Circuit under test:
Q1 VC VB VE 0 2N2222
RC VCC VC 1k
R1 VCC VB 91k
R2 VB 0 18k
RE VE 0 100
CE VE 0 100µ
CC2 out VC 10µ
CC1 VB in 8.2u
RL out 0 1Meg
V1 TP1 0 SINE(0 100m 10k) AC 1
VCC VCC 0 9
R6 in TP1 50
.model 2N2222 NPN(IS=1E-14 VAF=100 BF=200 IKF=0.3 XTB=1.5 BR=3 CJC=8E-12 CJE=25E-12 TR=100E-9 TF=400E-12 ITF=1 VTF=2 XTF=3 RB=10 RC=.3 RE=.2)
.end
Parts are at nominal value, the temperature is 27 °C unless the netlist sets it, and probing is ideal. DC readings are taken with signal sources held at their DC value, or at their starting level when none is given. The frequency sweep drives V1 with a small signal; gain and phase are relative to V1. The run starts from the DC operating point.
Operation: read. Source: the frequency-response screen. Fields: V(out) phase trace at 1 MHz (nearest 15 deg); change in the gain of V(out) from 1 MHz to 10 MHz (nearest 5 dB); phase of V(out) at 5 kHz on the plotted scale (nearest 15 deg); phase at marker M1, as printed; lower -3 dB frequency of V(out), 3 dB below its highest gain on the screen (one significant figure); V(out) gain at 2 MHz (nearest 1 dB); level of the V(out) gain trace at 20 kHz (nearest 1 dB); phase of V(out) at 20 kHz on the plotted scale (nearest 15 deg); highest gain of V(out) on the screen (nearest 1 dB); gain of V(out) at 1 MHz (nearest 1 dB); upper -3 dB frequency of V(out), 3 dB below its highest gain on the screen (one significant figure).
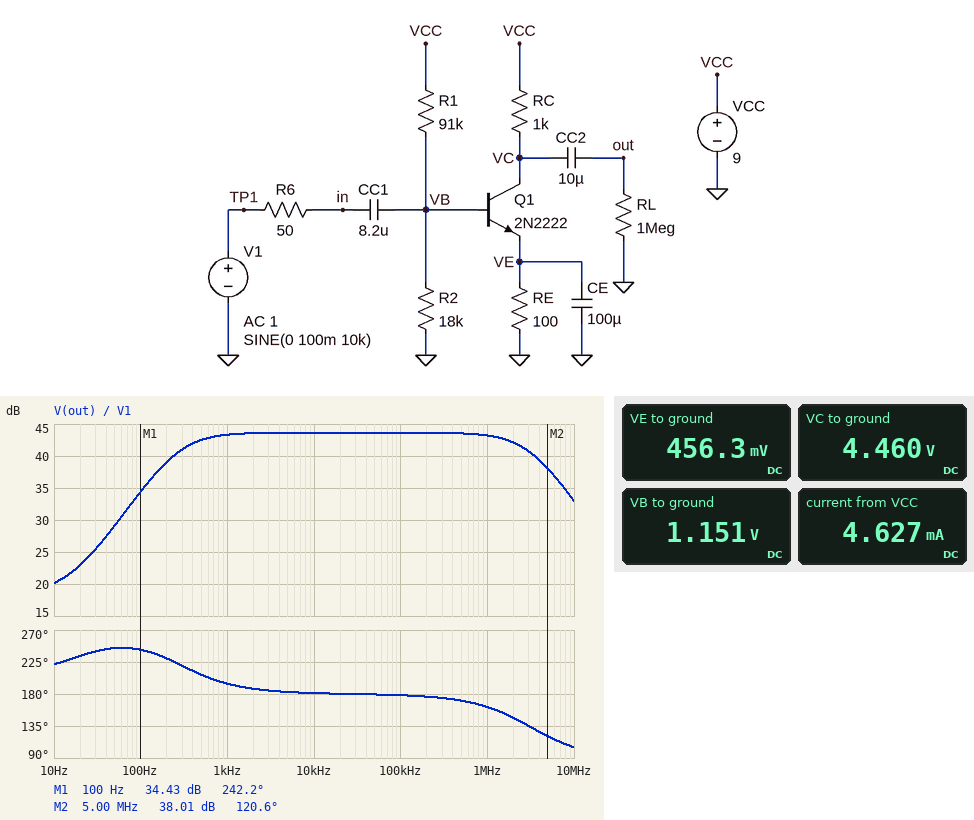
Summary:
165 deg
-10 dB
180 deg
242.2 deg
300 Hz
42 dB
44 dB
180 deg
44 dB
43 dB
3 MHz
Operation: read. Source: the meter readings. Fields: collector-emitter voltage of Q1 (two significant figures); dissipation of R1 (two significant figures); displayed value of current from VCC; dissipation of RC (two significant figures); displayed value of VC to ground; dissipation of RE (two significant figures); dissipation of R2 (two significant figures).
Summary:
4.0 V
680 µW
4.627 mA
21 mW
4.460 V
2.1 mW
74 µW
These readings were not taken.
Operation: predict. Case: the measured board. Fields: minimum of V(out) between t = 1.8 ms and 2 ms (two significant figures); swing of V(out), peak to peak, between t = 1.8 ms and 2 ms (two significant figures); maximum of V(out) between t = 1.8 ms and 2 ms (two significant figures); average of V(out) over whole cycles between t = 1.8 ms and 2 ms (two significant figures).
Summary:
-4.0 V
8.5 V
4.5 V
1.0 V
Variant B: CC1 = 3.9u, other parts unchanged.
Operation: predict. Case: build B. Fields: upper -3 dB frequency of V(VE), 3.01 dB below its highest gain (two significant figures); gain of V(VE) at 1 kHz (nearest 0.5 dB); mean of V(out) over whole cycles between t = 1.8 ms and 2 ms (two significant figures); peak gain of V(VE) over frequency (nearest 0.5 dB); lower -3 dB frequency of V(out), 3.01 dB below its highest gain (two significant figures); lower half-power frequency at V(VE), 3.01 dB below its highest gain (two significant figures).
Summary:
300 Hz
-12.5 dB
1.4 V
-1.5 dB
290 Hz
4.1 Hz
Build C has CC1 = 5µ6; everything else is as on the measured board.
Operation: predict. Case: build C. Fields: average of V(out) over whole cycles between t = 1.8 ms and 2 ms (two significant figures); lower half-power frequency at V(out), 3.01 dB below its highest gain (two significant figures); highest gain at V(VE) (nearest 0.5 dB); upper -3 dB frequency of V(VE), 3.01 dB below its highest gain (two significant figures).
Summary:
1.2 V
280 Hz
-1.5 dB
290 Hz
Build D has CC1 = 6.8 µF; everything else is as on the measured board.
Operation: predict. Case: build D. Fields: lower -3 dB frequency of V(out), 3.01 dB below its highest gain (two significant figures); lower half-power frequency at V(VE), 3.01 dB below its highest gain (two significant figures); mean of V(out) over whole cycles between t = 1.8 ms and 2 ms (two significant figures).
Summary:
280 Hz
2.5 Hz
1.1 V
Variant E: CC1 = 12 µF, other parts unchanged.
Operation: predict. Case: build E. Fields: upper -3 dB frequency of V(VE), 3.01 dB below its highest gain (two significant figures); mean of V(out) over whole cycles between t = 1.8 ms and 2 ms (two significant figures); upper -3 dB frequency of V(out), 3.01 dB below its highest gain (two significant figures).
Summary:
270 Hz
810 mV
3.1 MHz
